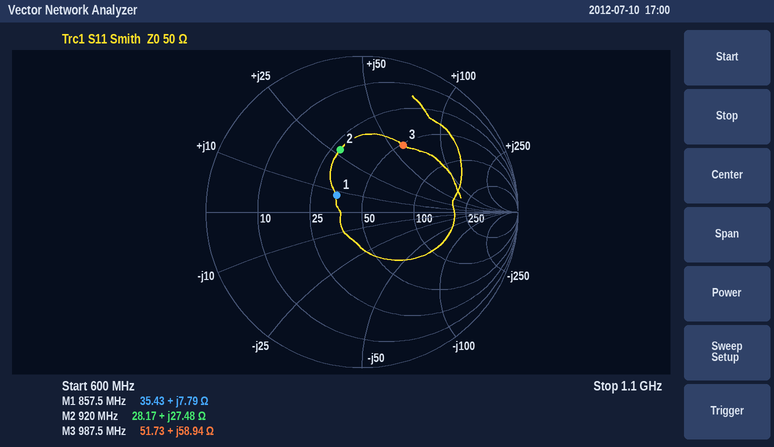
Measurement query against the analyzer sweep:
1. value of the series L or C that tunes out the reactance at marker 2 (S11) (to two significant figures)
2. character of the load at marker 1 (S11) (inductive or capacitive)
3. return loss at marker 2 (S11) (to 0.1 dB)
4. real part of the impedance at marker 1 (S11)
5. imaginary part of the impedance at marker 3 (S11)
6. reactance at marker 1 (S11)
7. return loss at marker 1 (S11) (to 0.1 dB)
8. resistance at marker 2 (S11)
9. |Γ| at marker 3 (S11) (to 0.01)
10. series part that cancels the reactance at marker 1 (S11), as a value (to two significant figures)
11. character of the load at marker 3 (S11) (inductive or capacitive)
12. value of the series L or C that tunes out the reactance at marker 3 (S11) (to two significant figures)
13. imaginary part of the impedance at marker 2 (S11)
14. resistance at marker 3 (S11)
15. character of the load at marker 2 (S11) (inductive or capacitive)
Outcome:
6.3 pF
inductive
7.5 dB
35.43 Ω
+58.94 Ω
+7.79 Ω
14.3 dB
28.17 Ω
0.50
24 pF
inductive
2.7 pF
+27.48 Ω
51.73 Ω
inductive
